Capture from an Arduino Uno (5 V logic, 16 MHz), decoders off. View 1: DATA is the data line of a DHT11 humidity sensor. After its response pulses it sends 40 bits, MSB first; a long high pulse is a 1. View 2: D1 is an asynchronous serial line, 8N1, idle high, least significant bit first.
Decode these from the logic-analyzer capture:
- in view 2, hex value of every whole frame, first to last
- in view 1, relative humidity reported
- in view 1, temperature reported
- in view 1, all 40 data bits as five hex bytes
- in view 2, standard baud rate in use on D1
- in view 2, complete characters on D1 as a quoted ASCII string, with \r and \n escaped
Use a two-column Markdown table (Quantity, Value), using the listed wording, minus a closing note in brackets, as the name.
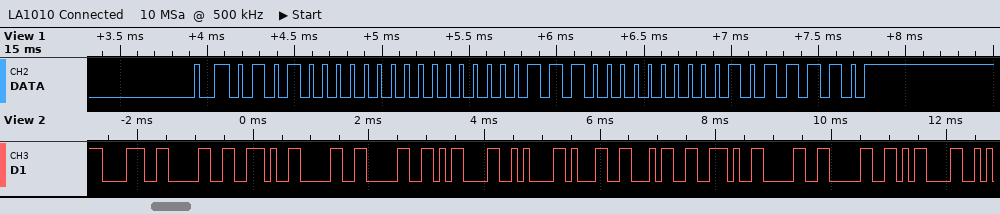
| Quantity | Value |
|---|---|
| in view 2, hex value of every whole frame, first to last | 38 30 2E 30 30 0D 0A 31 34 2E 30 30 0D |
| in view 1, relative humidity reported | 80 % |
| in view 1, temperature reported | 14.0 °C |
| in view 1, all 40 data bits as five hex bytes | 50 00 0E 00 5E |
| in view 2, standard baud rate in use on D1 | 9600 baud |
| in view 2, complete characters on D1 as a quoted ASCII string, with \r and \n escaped | "80.00\r\n14.00\r" |
